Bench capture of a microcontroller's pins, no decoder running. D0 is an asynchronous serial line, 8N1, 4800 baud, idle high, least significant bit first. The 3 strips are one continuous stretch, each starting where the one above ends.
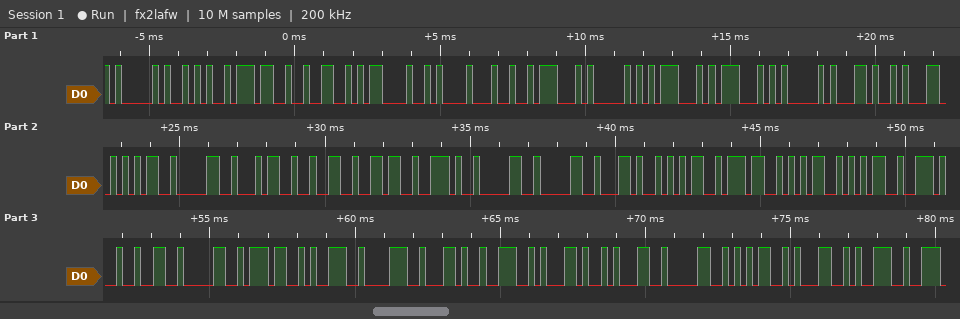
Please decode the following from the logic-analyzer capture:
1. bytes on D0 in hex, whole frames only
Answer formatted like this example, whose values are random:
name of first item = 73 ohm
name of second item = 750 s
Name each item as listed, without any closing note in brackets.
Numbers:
bytes on D0 in hex, whole frames only = 41 2A 37 32 0D 0A 24 47 50 47 47 41 2C 31 35 30 34 32 36 2E 30 30 2C 35 37 35 35 2E 32 30 37 39 38 2C 4E 2C 31 30 35 31 39
